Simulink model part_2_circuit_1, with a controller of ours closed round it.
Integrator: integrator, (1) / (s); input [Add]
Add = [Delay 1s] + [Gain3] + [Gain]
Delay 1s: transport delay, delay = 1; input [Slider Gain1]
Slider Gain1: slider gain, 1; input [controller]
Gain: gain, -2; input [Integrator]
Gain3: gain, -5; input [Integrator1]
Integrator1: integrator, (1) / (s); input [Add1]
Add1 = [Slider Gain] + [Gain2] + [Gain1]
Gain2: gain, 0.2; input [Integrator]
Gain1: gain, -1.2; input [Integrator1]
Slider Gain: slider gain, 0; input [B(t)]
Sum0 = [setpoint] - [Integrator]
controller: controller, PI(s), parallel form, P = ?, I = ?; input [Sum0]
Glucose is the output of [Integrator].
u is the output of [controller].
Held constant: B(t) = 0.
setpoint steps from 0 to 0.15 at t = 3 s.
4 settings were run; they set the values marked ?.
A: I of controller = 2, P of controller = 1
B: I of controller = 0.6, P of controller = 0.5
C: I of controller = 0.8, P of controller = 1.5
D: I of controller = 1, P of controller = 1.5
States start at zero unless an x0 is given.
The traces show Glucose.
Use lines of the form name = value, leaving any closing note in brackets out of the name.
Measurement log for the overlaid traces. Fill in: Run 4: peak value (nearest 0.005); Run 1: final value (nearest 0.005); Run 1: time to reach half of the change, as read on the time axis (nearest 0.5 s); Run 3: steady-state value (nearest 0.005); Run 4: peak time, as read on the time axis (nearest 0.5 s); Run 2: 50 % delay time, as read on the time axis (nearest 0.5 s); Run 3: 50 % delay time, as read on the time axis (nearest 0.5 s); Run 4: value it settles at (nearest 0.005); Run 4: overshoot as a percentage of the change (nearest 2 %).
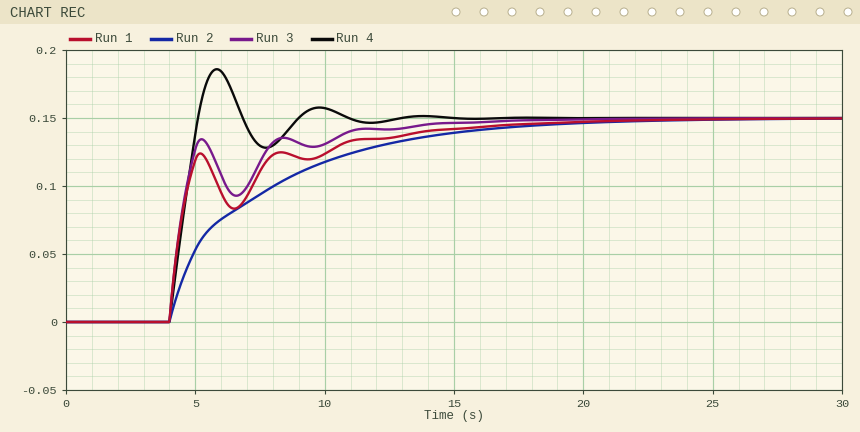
Run 4: peak value = 0.185
Run 1: final value = 0.150
Run 1: time to reach half of the change, as read on the time axis = 4.5 s
Run 3: steady-state value = 0.150
Run 4: peak time, as read on the time axis = 6.0 s
Run 2: 50 % delay time, as read on the time axis = 6.0 s
Run 3: 50 % delay time, as read on the time axis = 4.5 s
Run 4: value it settles at = 0.150
Run 4: overshoot as a percentage of the change = 24 %
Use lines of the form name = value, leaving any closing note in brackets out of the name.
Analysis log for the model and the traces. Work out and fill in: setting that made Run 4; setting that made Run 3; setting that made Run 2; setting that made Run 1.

setting that made Run 4 = A
setting that made Run 3 = D
setting that made Run 2 = B
setting that made Run 1 = C
